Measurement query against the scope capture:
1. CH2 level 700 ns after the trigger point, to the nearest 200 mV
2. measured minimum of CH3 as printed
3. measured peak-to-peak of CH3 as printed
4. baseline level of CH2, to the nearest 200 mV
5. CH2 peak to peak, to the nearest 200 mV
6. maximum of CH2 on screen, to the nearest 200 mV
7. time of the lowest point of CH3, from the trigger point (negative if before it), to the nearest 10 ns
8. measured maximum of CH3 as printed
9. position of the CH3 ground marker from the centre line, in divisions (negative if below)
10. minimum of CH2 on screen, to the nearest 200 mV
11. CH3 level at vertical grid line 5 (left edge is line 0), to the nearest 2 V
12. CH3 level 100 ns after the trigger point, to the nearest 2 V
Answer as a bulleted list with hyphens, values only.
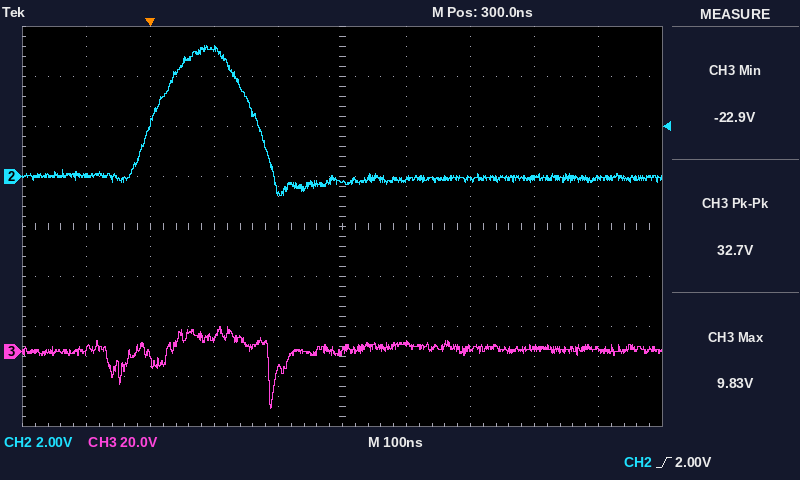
- 0.0 V
- -22.9 V
- 32.7 V
- 0.0 V
- 6.0 V
- 5.2 V
- +190 ns
- 9.83 V
- -2.5 div
- -800 mV
- 0 V
- 6 V
